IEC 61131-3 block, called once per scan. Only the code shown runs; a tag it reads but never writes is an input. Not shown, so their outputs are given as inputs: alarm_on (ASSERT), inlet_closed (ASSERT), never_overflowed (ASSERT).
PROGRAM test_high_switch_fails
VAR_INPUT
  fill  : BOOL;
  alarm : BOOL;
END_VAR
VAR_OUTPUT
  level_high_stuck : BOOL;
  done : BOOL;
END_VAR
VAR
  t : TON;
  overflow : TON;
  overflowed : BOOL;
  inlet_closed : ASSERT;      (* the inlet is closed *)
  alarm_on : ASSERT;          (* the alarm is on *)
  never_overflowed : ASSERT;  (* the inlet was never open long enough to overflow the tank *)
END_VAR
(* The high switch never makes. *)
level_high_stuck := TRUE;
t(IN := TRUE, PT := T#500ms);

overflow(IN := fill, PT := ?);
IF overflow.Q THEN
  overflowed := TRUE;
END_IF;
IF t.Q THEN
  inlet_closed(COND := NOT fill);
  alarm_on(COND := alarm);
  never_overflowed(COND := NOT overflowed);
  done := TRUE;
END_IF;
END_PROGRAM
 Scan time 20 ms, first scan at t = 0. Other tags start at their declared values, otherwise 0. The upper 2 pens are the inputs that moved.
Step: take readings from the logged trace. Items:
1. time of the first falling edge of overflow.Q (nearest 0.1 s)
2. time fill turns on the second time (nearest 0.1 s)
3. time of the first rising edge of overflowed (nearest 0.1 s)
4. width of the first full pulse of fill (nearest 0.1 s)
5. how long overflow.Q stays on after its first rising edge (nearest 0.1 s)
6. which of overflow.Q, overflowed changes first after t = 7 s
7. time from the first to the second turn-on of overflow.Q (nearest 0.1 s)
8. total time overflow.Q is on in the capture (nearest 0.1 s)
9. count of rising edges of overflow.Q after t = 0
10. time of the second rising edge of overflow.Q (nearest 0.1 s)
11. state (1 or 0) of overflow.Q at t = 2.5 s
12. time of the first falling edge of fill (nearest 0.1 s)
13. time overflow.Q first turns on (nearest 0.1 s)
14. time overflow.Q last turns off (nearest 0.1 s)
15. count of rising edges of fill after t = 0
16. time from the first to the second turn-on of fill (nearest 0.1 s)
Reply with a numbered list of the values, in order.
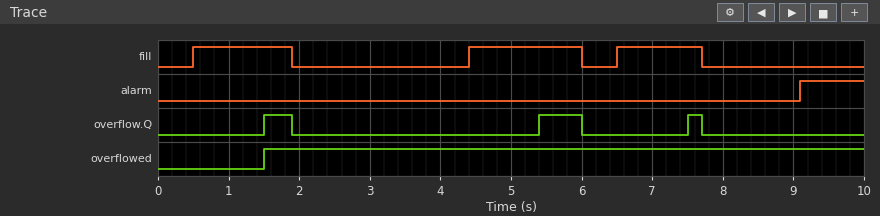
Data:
1. 1.9 s
2. 4.4 s
3. 1.5 s
4. 1.4 s
5. 0.4 s
6. overflow.Q
7. 3.9 s
8. 1.2 s
9. 3
10. 5.4 s
11. 0
12. 1.9 s
13. 1.5 s
14. 7.7 s
15. 3
16. 3.9 s
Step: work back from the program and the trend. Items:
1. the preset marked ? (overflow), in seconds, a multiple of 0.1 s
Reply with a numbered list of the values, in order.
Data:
1. 1.0 s
